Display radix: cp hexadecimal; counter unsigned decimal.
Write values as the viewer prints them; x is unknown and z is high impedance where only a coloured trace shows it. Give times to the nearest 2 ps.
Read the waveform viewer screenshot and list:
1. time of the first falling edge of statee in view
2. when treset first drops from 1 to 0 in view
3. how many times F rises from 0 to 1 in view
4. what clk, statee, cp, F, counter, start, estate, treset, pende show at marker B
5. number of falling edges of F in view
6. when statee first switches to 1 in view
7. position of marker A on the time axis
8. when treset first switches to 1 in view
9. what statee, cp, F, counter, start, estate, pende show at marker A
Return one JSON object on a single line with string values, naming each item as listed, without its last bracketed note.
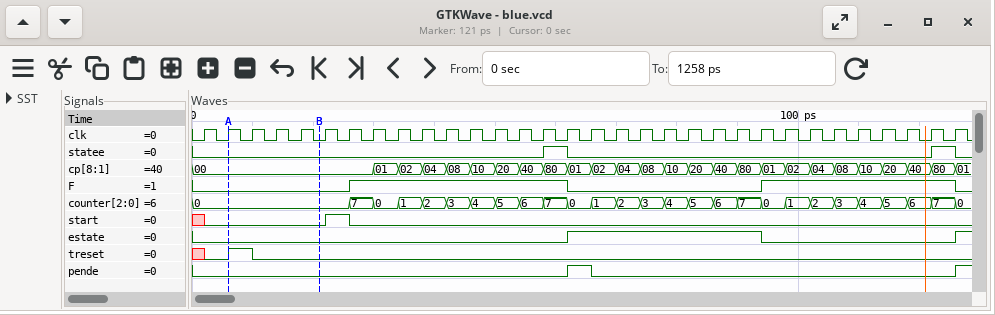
{"time of the first falling edge of statee in view": "62 ps", "when treset first drops from 1 to 0 in view": "10 ps", "how many times F rises from 0 to 1 in view": "2", "what clk, statee, cp, F, counter, start, estate, treset, pende show at marker B": "clk=0, statee=0, cp=00, F=0, counter=0, start=0, estate=0, treset=0, pende=0", "number of falling edges of F in view": "2", "when statee first switches to 1 in view": "58 ps", "position of marker A on the time axis": "6 ps", "when treset first switches to 1 in view": "6 ps", "what statee, cp, F, counter, start, estate, pende show at marker A": "statee=0, cp=00, F=0, counter=0, start=0, estate=0, pende=0"}
